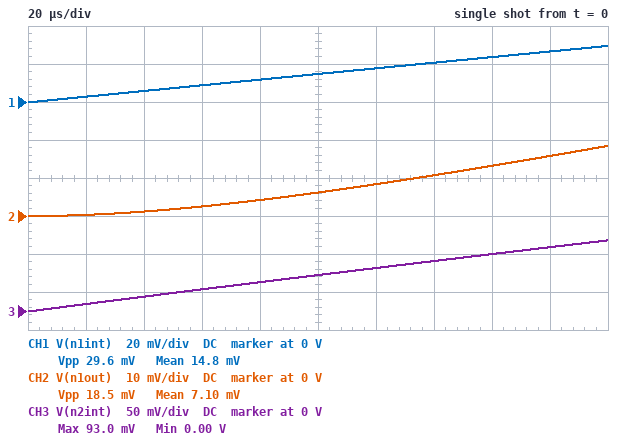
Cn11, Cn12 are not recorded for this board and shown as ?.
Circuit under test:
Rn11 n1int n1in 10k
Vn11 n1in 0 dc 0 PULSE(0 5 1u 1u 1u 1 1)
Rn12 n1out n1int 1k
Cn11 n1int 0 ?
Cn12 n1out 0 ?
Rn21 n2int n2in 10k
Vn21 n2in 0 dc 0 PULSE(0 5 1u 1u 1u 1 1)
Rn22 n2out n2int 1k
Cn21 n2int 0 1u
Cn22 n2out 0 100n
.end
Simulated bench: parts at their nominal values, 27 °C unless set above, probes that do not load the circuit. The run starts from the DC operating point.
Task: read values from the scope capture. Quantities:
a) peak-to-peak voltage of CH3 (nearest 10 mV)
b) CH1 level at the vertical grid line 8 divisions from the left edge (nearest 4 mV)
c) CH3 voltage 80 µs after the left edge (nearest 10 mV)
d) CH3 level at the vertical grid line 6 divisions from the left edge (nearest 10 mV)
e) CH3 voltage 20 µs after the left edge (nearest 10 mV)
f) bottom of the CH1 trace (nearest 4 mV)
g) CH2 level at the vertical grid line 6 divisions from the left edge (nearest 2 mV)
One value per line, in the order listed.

90 mV
24 mV
40 mV
60 mV
10 mV
0 V
8 mV
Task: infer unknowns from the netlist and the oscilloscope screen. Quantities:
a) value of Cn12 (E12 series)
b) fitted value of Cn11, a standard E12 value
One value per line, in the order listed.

82 nF
3.3 µF
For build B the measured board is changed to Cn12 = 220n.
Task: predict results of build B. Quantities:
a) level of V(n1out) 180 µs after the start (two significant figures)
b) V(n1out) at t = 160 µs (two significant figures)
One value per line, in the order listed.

8.4 mV
6.8 mV
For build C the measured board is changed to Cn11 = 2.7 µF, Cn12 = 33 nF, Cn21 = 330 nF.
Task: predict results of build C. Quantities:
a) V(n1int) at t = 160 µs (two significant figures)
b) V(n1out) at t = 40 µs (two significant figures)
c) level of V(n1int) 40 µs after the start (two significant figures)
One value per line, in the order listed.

29 mV
2.9 mV
7.1 mV
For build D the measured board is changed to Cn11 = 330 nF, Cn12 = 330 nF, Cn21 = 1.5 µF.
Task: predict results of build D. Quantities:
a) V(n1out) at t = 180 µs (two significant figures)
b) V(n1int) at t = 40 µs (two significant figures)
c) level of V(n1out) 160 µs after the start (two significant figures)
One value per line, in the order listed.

52 mV
55 mV
42 mV
